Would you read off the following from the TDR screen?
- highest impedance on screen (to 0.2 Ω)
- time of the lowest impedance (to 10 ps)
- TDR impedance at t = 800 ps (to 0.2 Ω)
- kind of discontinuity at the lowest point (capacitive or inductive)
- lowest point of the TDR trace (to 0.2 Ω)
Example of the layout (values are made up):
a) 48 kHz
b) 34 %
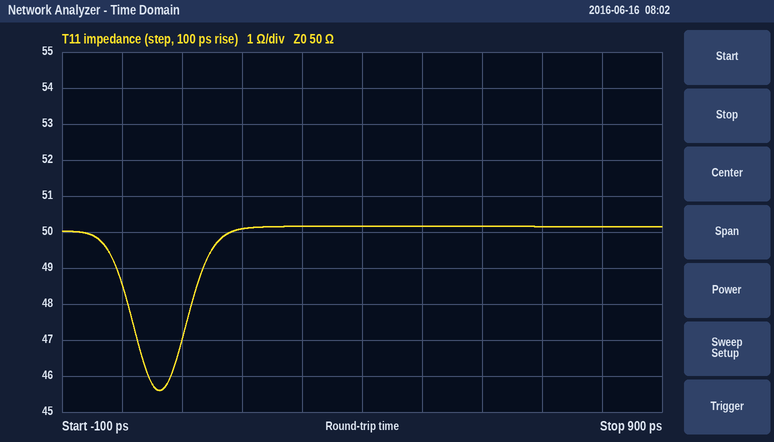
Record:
a) 50.2 Ω
b) 60 ps
c) 50.2 Ω
d) capacitive
e) 45.6 Ω
